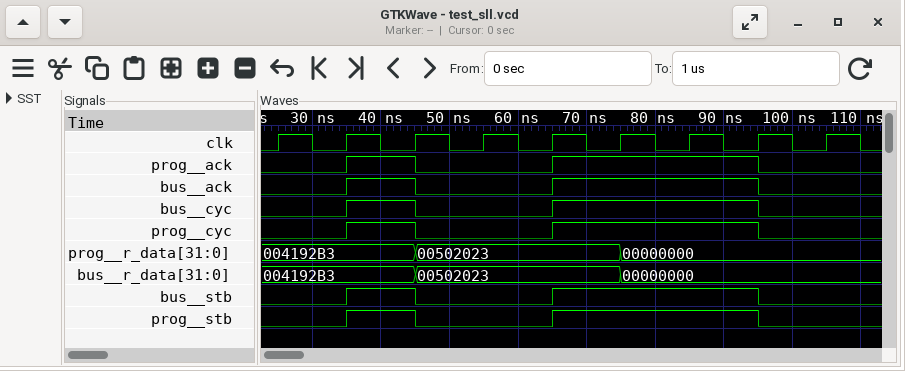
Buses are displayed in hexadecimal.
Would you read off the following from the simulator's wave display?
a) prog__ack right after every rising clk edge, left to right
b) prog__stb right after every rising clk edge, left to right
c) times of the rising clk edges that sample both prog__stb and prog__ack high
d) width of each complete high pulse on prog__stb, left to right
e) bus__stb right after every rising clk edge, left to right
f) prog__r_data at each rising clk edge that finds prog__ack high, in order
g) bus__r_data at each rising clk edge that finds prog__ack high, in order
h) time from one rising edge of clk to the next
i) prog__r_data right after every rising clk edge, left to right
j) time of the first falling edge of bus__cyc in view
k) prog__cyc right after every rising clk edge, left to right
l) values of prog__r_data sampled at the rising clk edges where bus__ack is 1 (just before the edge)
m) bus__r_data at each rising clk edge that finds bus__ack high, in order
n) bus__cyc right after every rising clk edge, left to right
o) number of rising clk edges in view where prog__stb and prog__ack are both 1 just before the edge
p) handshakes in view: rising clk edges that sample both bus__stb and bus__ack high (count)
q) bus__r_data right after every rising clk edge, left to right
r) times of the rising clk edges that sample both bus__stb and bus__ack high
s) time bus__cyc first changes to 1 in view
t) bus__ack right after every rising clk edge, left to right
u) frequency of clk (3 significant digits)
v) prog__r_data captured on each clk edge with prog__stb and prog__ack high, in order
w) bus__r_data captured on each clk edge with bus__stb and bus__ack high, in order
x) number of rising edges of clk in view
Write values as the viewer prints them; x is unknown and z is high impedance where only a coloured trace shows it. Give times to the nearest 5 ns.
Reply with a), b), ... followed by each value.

a) 0 1 0 0 1 1 1 0 0
b) 0 1 0 0 1 1 1 0 0
c) 45 ns, 75 ns, 85 ns, 95 ns
d) 10 ns, 30 ns
e) 0 1 0 0 1 1 1 0 0
f) 004192B3, 00502023, 00000000, 00000000
g) 004192B3, 00502023, 00000000, 00000000
h) 10 ns
i) 004192B3, 004192B3, 00502023, 00502023, 00502023, 00000000, 00000000, 00000000, 00000000
j) 45 ns
k) 0 1 0 0 1 1 1 0 0
l) 004192B3, 00502023, 00000000, 00000000
m) 004192B3, 00502023, 00000000, 00000000
n) 0 1 0 0 1 1 1 0 0
o) 4
p) 4
q) 004192B3, 004192B3, 00502023, 00502023, 00502023, 00000000, 00000000, 00000000, 00000000
r) 45 ns, 75 ns, 85 ns, 95 ns
s) 35 ns
t) 0 1 0 0 1 1 1 0 0
u) 100 MHz
v) 004192B3, 00502023, 00000000, 00000000
w) 004192B3, 00502023, 00000000, 00000000
x) 9
